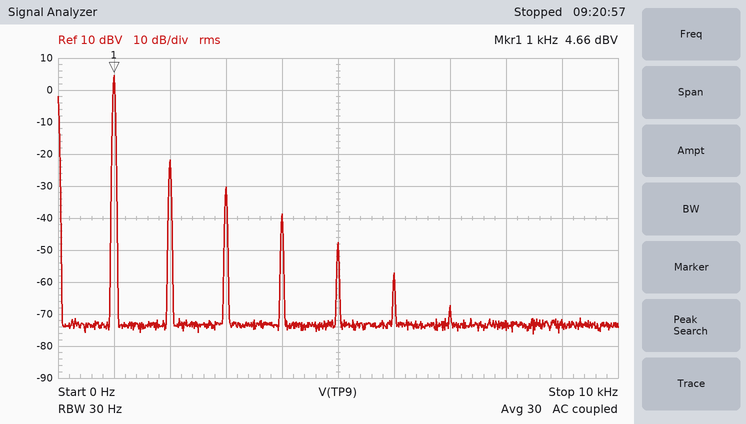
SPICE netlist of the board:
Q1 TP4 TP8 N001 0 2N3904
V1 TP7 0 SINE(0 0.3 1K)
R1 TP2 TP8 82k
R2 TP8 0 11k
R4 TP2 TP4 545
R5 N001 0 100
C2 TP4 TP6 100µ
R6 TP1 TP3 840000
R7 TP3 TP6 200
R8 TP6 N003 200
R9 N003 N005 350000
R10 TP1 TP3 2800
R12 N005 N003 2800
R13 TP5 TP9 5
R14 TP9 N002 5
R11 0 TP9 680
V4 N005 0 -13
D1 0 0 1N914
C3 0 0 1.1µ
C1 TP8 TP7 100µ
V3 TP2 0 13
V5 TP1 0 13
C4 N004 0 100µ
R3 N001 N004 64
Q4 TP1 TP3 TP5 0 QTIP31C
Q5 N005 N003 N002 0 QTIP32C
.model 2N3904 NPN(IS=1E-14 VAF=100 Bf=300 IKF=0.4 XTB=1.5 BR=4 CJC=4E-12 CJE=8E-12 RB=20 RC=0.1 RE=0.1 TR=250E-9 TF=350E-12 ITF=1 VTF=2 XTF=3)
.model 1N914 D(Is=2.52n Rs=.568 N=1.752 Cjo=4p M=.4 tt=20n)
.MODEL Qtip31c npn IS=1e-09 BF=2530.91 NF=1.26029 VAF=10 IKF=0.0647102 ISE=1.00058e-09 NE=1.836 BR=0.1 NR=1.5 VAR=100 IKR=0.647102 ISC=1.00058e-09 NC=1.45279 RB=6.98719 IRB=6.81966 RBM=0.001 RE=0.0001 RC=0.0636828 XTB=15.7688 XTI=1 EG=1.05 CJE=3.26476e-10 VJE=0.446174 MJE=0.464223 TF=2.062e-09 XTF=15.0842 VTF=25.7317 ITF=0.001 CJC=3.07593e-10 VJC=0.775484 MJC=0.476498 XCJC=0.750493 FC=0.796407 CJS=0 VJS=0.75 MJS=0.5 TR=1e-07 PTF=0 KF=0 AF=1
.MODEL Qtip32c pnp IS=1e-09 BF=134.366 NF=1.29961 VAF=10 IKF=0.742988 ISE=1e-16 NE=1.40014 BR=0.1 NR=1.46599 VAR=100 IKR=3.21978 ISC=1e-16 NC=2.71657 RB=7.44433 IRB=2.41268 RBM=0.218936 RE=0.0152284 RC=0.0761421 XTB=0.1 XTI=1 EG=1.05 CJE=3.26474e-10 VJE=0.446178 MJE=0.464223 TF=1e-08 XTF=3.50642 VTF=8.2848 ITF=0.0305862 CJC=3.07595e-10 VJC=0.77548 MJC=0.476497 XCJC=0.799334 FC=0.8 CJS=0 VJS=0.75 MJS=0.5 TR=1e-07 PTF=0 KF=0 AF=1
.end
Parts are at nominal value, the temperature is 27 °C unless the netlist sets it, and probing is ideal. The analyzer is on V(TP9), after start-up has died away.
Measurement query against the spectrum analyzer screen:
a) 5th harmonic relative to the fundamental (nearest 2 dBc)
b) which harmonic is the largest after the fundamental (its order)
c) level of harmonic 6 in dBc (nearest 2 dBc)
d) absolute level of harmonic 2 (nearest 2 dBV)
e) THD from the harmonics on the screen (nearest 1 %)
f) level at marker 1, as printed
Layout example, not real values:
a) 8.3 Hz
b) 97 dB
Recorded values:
a) -52 dBc
b) 2
c) -62 dBc
d) -22 dBV
e) 5 %
f) 4.66 dBV
